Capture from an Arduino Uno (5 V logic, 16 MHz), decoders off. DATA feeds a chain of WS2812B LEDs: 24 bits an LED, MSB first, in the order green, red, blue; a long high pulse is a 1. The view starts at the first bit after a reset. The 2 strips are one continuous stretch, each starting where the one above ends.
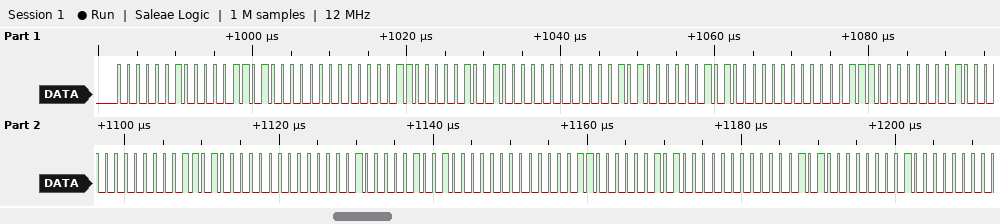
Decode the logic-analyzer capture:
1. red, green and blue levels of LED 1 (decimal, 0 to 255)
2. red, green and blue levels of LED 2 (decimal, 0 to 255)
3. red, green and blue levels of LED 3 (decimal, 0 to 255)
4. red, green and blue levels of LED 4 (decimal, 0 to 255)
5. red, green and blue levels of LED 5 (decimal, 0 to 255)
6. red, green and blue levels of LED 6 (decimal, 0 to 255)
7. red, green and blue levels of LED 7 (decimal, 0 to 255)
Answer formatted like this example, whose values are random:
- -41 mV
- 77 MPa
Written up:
- 13, 2, 0
- 9, 6, 0
- 5, 10, 0
- 1, 14, 0
- 0, 13, 2
- 0, 9, 6
- 0, 5, 10
